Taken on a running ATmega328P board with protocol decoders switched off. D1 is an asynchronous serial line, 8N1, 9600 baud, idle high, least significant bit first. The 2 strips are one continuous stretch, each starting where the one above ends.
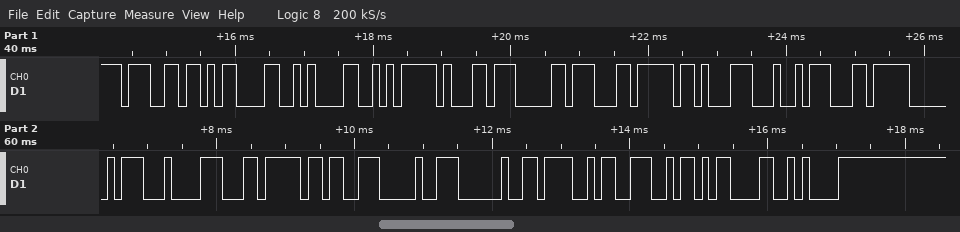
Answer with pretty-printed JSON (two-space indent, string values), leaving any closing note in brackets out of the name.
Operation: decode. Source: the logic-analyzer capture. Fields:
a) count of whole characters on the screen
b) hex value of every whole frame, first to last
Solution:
{
  "count of whole characters on the screen": "20",
  "hex value of every whole frame, first to last": "0x67 0x0D 0x0A 0xEA 0xB1 0xB0 0xEC 0x8B 0xA4 0xEC 0xA0 0x84 0xEC 0x9B 0x90 0x20 0x4F 0x4E 0x0D 0x0A"
}
